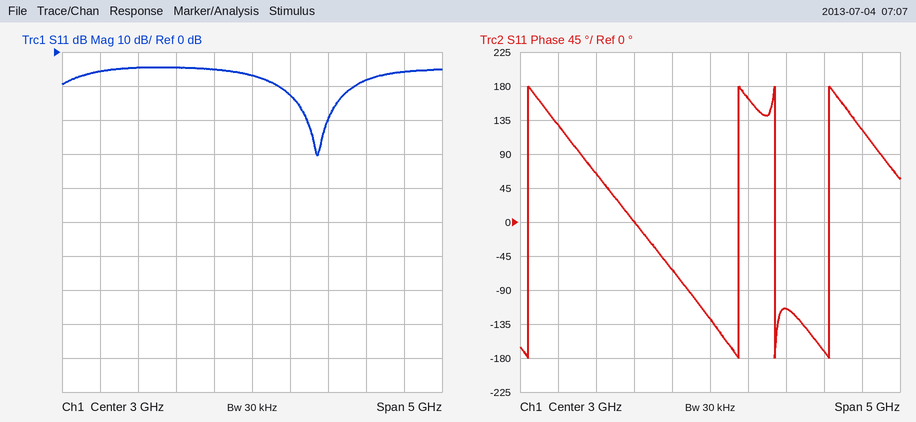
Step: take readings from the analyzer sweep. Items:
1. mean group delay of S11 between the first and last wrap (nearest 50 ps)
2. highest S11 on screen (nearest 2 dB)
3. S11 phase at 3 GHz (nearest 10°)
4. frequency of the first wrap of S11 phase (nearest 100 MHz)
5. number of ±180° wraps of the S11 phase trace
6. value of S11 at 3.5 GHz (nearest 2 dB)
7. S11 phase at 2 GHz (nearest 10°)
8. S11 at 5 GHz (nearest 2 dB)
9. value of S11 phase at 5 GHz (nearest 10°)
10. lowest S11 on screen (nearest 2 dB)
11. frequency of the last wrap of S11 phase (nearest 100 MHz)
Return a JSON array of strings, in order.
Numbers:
["750 ps", "-4 dB", "-130°", "600 MHz", "4", "-12 dB", "0°", "-6 dB", "120°", "-30 dB", "4.6 GHz"]
